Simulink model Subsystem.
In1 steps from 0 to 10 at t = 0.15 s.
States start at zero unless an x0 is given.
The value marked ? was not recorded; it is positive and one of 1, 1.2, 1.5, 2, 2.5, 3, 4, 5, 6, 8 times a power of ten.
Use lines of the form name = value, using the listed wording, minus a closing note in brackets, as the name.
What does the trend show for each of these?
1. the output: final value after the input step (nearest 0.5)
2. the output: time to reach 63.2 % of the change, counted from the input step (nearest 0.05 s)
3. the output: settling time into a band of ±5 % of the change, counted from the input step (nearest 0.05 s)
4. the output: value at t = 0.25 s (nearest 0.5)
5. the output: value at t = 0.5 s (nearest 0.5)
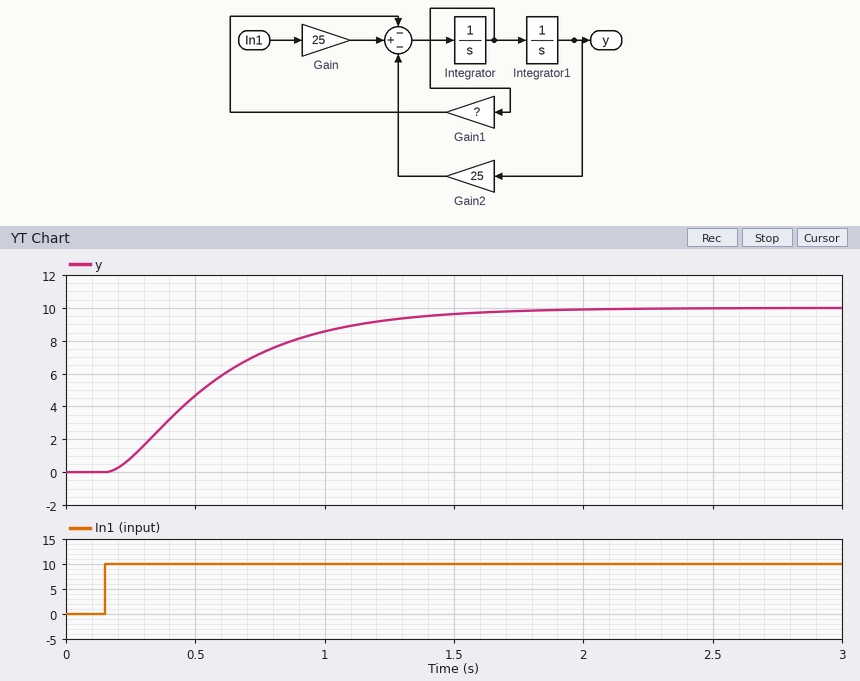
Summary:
the output: final value after the input step = 10.0
the output: time to reach 63.2 % of the change, counted from the input step = 0.50 s
the output: settling time into a band of ±5 % of the change, counted from the input step = 1.25 s
the output: value at t = 0.25 s = 1.0
the output: value at t = 0.5 s = 4.5
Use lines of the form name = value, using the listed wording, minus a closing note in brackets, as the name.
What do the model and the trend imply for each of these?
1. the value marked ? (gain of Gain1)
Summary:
the value marked ? = 12
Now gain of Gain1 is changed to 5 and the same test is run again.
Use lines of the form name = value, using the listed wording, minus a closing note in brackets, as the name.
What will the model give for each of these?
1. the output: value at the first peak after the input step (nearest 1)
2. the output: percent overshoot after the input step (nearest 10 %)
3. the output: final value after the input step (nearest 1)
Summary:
the output: value at the first peak after the input step = 12
the output: percent overshoot after the input step = 20 %
the output: final value after the input step = 10
